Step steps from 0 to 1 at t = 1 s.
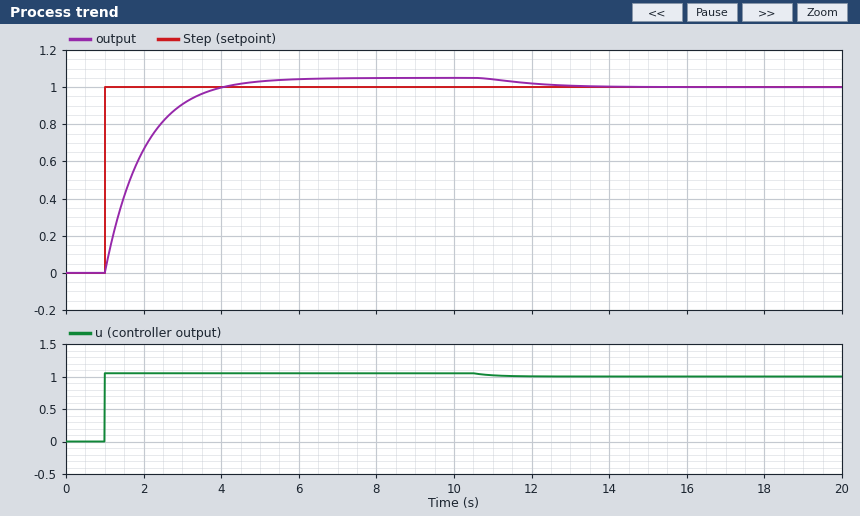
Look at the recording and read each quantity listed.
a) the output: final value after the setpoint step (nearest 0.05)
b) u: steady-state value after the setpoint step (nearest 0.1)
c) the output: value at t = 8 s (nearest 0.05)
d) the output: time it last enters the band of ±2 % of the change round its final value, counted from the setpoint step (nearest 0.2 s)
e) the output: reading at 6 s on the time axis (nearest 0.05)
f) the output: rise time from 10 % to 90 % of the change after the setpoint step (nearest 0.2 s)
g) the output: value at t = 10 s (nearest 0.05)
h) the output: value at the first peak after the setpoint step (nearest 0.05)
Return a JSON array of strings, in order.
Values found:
["1.00", "1.0", "1.05", "11.0 s", "1.05", "1.8 s", "1.05", "1.05"]
